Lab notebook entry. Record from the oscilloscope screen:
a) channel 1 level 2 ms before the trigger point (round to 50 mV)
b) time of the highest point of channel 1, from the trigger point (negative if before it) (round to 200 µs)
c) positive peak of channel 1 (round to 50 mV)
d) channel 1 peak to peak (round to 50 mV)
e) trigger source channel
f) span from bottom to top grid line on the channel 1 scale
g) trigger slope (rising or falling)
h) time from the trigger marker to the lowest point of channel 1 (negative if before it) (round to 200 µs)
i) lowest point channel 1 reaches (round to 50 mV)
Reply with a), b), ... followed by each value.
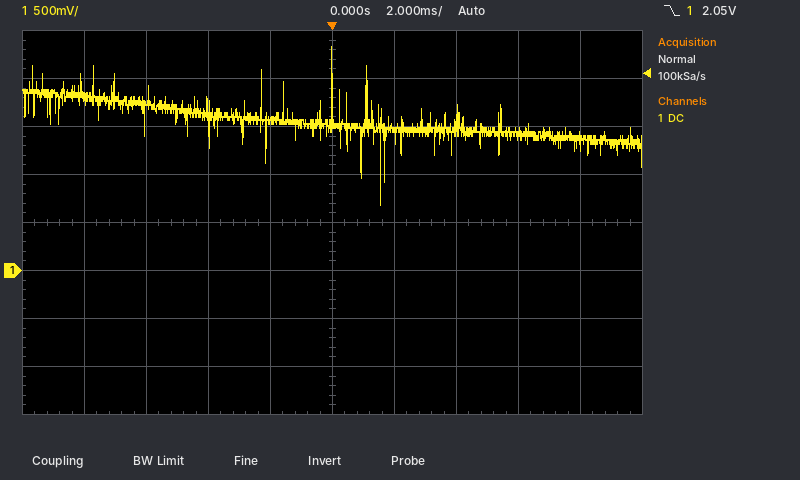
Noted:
a) 1.55 V
b) 0.0 ms
c) 2.35 V
d) 1.65 V
e) channel 1
f) 4 V
g) falling
h) +1.6 ms
i) 700 mV
